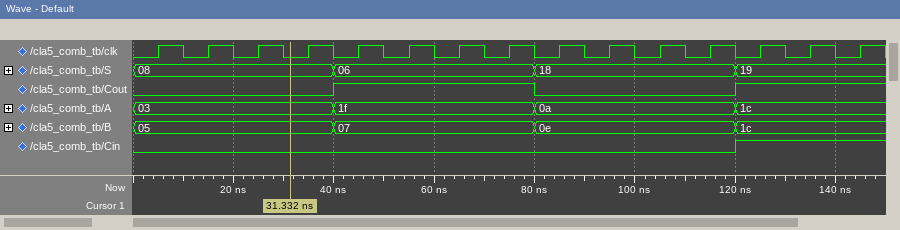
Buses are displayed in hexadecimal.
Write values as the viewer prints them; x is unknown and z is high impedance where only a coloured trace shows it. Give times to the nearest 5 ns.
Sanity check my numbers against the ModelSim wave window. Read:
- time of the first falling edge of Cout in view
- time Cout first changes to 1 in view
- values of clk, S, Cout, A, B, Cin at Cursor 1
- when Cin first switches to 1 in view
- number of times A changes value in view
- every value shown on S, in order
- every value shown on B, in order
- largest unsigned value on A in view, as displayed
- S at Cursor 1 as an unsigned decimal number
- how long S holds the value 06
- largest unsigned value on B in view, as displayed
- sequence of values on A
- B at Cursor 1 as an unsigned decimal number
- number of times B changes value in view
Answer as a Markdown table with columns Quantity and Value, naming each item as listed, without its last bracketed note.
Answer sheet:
| Quantity | Value |
|---|---|
| time of the first falling edge of Cout in view | 80 ns |
| time Cout first changes to 1 in view | 40 ns |
| values of clk, S, Cout, A, B, Cin at Cursor 1 | clk=0, S=08, Cout=0, A=03, B=05, Cin=0 |
| when Cin first switches to 1 in view | 120 ns |
| number of times A changes value in view | 3 |
| every value shown on S, in order | 08, 06, 18, 19 |
| every value shown on B, in order | 05, 07, 0e, 1c |
| largest unsigned value on A in view, as displayed | 1f |
| S at Cursor 1 as an unsigned decimal number | 8 |
| how long S holds the value 06 | 40 ns |
| largest unsigned value on B in view, as displayed | 1c |
| sequence of values on A | 03, 1f, 0a, 1c |
| B at Cursor 1 as an unsigned decimal number | 5 |
| number of times B changes value in view | 3 |
